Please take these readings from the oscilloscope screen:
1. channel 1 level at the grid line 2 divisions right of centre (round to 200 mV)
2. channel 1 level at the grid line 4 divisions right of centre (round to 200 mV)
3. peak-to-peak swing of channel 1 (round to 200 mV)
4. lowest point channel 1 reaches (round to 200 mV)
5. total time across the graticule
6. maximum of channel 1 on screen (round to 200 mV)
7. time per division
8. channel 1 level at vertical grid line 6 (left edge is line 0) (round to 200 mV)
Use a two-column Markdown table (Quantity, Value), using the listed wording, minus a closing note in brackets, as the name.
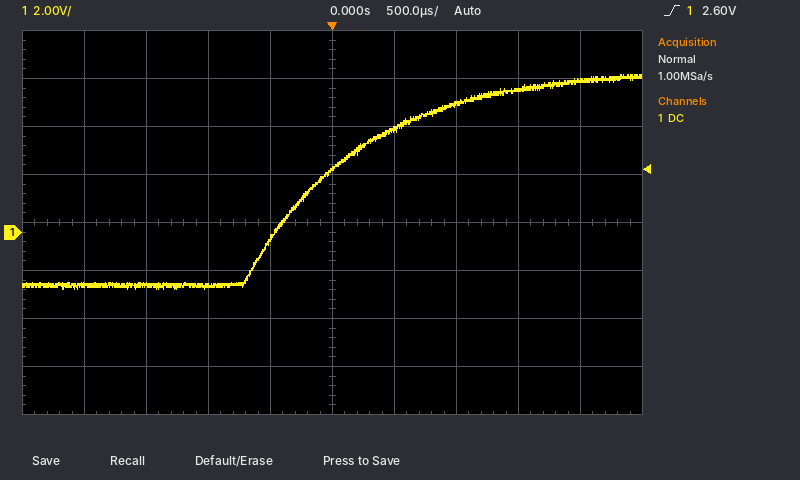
| Quantity | Value |
|---|---|
| channel 1 level at the grid line 2 divisions right of centre | 5.4 V |
| channel 1 level at the grid line 4 divisions right of centre | 6.4 V |
| peak-to-peak swing of channel 1 | 9.0 V |
| lowest point channel 1 reaches | -2.4 V |
| total time across the graticule | 5 ms |
| maximum of channel 1 on screen | 6.6 V |
| time per division | 500 µs |
| channel 1 level at vertical grid line 6 (left edge is line 0) | 4.2 V |
